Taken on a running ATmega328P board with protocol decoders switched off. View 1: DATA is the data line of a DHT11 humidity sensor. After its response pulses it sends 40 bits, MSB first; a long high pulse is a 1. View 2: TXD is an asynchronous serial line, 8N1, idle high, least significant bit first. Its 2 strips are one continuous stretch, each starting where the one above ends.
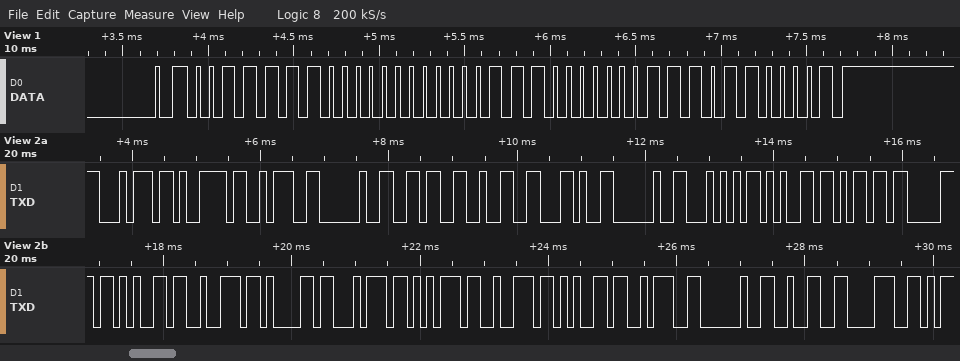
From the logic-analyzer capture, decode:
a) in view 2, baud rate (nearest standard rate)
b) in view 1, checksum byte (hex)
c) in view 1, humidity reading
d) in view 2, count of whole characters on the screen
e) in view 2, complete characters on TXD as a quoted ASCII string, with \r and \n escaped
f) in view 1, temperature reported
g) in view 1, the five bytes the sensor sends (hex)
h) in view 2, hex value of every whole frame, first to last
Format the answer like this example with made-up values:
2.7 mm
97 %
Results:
9600 baud
0x61
62 %
23
"ty: 62, Temperature: 28"
28.7 °C
3E 00 1C 07 61
74 79 3A 20 36 32 2C 20 54 65 6D 70 65 72 61 74 75 72 65 3A 20 32 38
